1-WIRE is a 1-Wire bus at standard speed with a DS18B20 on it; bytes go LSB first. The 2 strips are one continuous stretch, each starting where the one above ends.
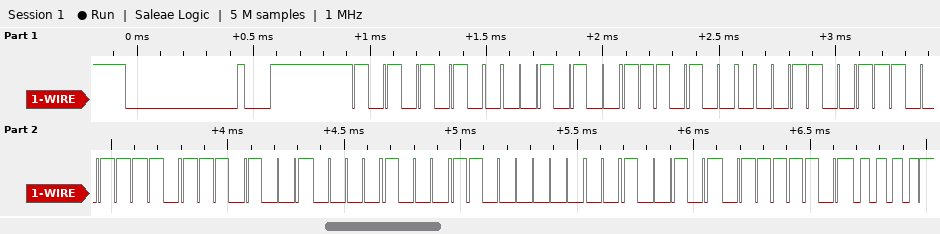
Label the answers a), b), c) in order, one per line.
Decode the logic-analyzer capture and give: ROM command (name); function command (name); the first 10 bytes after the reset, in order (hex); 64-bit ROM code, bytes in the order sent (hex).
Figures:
a) Match ROM
b) Read Scratchpad
c) 55 28 17 CC 79 97 10 03 A4 BE
d) 28 17 CC 79 97 10 03 A4
